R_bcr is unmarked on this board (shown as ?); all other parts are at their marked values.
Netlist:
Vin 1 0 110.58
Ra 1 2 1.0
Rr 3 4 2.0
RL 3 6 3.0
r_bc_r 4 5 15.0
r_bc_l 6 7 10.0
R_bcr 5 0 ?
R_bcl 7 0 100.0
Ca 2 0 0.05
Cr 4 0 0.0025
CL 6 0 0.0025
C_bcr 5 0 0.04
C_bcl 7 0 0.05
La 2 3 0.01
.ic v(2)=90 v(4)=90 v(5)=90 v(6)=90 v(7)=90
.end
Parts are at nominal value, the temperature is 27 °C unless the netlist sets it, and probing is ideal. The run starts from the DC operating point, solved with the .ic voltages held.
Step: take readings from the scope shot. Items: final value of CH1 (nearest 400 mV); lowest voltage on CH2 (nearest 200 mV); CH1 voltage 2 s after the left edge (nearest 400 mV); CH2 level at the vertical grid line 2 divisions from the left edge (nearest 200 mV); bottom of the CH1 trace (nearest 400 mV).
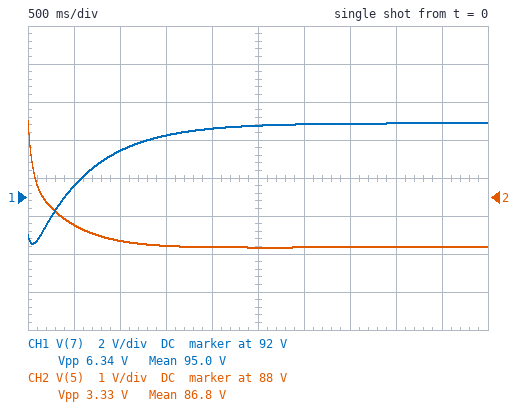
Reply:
96.0 V
86.6 V
95.6 V
86.8 V
89.6 V
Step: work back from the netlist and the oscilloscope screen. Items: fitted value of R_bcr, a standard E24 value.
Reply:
68 Ω
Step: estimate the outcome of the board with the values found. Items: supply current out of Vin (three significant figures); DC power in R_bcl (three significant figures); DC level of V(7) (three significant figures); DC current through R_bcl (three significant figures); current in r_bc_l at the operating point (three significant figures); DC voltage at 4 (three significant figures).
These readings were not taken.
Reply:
2.23 A
91.9 W
95.9 V
959 mA
959 mA
106 V
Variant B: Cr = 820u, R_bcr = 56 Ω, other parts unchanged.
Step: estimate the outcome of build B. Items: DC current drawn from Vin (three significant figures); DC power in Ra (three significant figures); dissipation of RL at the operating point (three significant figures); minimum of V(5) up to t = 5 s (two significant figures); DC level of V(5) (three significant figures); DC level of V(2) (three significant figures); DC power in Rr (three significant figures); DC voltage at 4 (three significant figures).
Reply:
2.44 A
5.95 W
2.75 W
83 V
83.0 V
108 V
4.39 W
105 V
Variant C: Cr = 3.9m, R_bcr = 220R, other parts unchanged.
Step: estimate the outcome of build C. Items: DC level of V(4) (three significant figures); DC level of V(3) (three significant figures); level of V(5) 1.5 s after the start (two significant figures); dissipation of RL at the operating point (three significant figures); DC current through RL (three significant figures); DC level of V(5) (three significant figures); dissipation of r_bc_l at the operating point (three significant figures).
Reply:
108 V
109 V
100 V
2.80 W
966 mA
101 V
9.33 W
